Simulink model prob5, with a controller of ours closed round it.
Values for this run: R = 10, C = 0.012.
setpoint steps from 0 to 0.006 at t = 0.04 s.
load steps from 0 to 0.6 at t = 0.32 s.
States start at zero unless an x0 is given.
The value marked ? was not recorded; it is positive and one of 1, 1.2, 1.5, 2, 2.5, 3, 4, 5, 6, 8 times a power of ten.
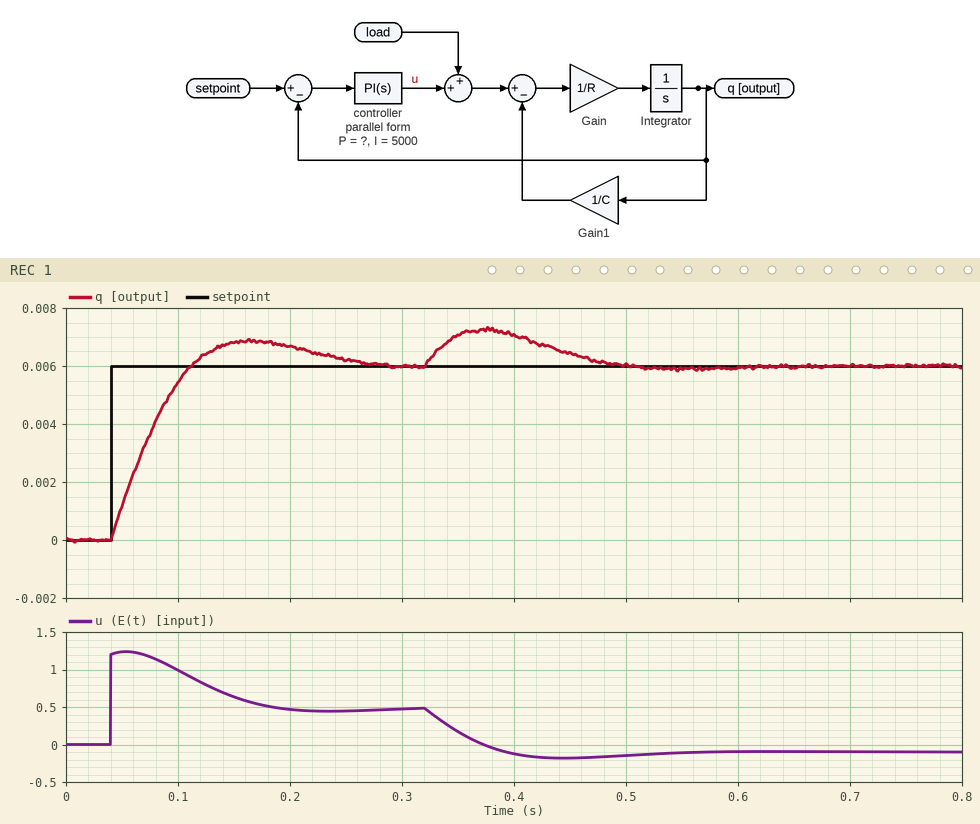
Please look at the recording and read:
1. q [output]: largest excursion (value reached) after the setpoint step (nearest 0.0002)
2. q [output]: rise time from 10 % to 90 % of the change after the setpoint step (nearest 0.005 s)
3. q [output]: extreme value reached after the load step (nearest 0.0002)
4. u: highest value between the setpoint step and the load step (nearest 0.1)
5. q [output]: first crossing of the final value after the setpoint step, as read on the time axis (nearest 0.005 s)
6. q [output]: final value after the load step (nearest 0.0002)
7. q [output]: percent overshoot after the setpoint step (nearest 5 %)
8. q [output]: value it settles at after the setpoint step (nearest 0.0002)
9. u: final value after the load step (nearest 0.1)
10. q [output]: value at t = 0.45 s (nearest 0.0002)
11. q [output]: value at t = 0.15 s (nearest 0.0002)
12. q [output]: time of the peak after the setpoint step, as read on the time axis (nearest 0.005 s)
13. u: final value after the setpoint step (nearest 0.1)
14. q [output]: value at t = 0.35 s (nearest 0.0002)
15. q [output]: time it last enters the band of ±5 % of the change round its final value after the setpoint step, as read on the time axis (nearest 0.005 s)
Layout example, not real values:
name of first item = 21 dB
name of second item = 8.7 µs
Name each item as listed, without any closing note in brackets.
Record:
q [output]: largest excursion (value reached) after the setpoint step = 0.0068
q [output]: rise time from 10 % to 90 % of the change after the setpoint step = 0.055 s
q [output]: extreme value reached after the load step = 0.0072
u: highest value between the setpoint step and the load step = 1.2
q [output]: first crossing of the final value after the setpoint step, as read on the time axis = 0.110 s
q [output]: final value after the load step = 0.0060
q [output]: percent overshoot after the setpoint step = 15 %
q [output]: value it settles at after the setpoint step = 0.0060
u: final value after the load step = -0.1
q [output]: value at t = 0.45 s = 0.0064
q [output]: value at t = 0.15 s = 0.0068
q [output]: time of the peak after the setpoint step, as read on the time axis = 0.165 s
u: final value after the setpoint step = 0.5
q [output]: value at t = 0.35 s = 0.0070
q [output]: time it last enters the band of ±5 % of the change round its final value after the setpoint step, as read on the time axis = 0.240 s
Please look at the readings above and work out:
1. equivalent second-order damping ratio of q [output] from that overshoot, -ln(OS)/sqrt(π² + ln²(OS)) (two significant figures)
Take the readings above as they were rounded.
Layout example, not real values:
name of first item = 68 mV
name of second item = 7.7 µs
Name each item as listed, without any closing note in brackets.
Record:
equivalent second-order damping ratio of q [output] from that overshoot, -ln(OS)/sqrt(π² + ln²(OS)) = 0.52
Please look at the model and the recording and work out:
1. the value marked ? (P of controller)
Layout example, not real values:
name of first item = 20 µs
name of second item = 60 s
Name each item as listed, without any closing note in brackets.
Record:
the value marked ? = 200
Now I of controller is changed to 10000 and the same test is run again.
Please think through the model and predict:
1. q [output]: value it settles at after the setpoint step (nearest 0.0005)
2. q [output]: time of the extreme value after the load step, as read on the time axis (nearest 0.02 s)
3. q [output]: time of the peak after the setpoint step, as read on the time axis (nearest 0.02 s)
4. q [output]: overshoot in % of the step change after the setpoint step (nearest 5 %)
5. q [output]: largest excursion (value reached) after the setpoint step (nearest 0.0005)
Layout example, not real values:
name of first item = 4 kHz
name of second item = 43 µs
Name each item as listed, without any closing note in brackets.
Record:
q [output]: value it settles at after the setpoint step = 0.0060
q [output]: time of the extreme value after the load step, as read on the time axis = 0.36 s
q [output]: time of the peak after the setpoint step, as read on the time axis = 0.12 s
q [output]: overshoot in % of the step change after the setpoint step = 25 %
q [output]: largest excursion (value reached) after the setpoint step = 0.0075
